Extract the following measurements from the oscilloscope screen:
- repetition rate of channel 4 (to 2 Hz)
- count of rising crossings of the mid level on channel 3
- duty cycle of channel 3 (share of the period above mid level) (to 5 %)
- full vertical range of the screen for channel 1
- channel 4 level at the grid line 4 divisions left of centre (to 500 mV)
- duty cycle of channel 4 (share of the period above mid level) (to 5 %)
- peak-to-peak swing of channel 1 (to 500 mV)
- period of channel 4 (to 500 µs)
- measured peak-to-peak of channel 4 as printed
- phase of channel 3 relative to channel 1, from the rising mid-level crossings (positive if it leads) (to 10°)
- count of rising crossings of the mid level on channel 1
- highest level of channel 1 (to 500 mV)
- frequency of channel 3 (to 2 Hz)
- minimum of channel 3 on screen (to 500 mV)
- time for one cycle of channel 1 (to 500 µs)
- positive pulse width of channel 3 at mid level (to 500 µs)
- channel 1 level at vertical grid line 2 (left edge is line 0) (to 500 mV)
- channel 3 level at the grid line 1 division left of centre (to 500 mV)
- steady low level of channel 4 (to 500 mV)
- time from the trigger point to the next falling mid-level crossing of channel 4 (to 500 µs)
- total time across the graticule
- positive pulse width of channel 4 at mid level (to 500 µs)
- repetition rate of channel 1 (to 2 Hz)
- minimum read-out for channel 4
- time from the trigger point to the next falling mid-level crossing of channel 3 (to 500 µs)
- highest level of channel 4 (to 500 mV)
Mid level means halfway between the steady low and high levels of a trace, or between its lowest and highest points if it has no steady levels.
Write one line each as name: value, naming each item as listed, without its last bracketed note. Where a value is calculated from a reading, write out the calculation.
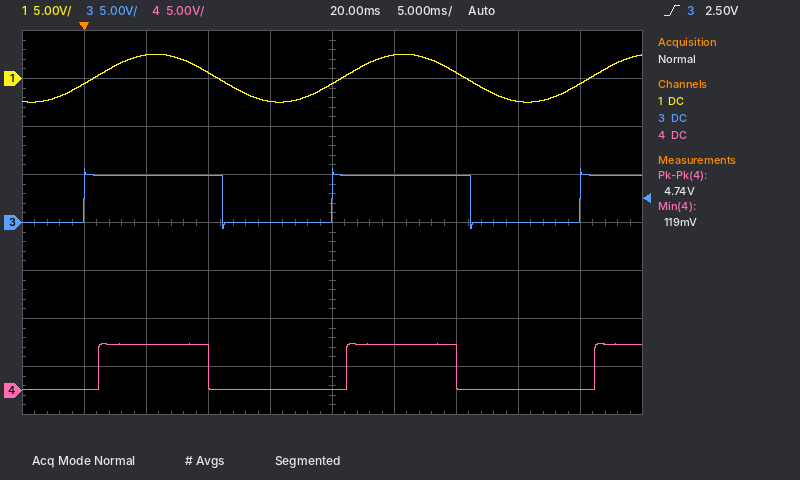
repetition rate of channel 4: 1 / 20.0 ms ≈ 50 Hz
count of rising crossings of the mid level on channel 3: 3
duty cycle of channel 3 (share of the period above mid level): 11.0 ms / 20.0 ms ≈ 55 %
full vertical range of the screen for channel 1: 40 V
channel 4 level at the grid line 4 divisions left of centre: 0.0 V
duty cycle of channel 4 (share of the period above mid level): 9.0 ms / 20.0 ms ≈ 45 %
peak-to-peak swing of channel 1: 2.5 V − (-2.5 V) = 5.0 V
period of channel 4: 20.0 ms
measured peak-to-peak of channel 4 as printed: 4.74 V
phase of channel 3 relative to channel 1, from the rising mid-level crossings (positive if it leads): +10°
count of rising crossings of the mid level on channel 1: 3
highest level of channel 1: 2.5 V
frequency of channel 3: 1 / 20.0 ms ≈ 50 Hz
minimum of channel 3 on screen: -500 mV
time for one cycle of channel 1: 20.0 ms
positive pulse width of channel 3 at mid level: 11.0 ms
channel 1 level at vertical grid line 2 (left edge is line 0): 2.5 V
channel 3 level at the grid line 1 division left of centre: 0.0 V
steady low level of channel 4: 0.0 V
time from the trigger point to the next falling mid-level crossing of channel 4: 10.0 ms
total time across the graticule: 50 ms
positive pulse width of channel 4 at mid level: 9.0 ms
repetition rate of channel 1: 1 / 20.0 ms ≈ 50 Hz
minimum read-out for channel 4: 119 mV
time from the trigger point to the next falling mid-level crossing of channel 3: 11.0 ms
highest level of channel 4: 5.0 V
